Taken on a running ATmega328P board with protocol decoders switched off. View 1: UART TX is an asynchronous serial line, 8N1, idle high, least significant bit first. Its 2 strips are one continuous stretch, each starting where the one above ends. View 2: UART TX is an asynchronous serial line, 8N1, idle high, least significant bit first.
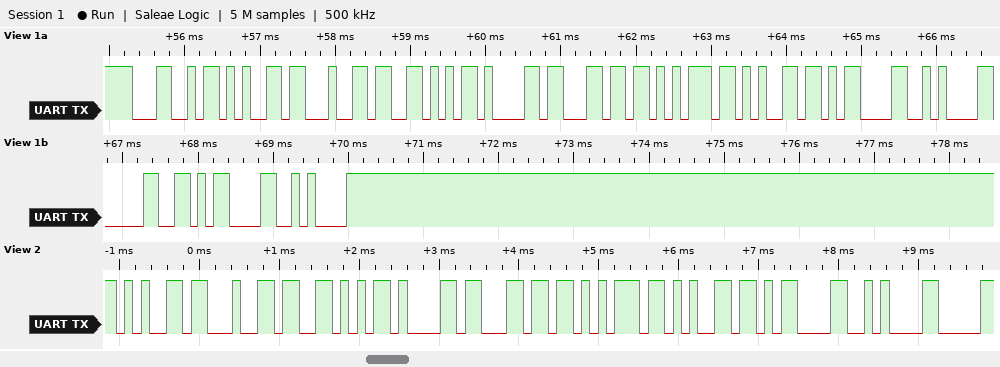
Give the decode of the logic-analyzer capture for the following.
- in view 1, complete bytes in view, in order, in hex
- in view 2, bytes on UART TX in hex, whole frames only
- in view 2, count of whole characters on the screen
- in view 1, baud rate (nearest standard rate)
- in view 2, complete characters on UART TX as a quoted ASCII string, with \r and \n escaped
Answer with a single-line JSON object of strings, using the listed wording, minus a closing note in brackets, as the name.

{"in view 1, complete bytes in view, in order, in hex": "4C 65 64 56 61 6C 75 65 0D 0A 30 0D 0A", "in view 2, bytes on UART TX in hex, whole frames only": "65 64 56 61 6C 75 65 0D 0A", "in view 2, count of whole characters on the screen": "9", "in view 1, baud rate": "9600 baud", "in view 2, complete characters on UART TX as a quoted ASCII string, with \\r and \\n escaped": "\"edValue\\r\\n\""}
